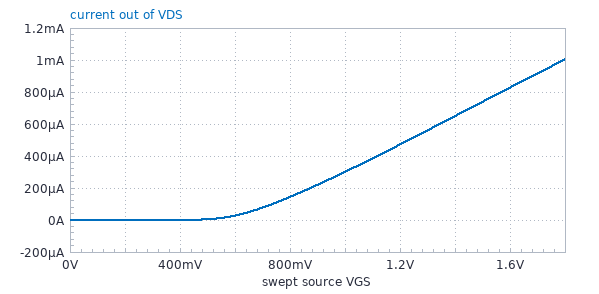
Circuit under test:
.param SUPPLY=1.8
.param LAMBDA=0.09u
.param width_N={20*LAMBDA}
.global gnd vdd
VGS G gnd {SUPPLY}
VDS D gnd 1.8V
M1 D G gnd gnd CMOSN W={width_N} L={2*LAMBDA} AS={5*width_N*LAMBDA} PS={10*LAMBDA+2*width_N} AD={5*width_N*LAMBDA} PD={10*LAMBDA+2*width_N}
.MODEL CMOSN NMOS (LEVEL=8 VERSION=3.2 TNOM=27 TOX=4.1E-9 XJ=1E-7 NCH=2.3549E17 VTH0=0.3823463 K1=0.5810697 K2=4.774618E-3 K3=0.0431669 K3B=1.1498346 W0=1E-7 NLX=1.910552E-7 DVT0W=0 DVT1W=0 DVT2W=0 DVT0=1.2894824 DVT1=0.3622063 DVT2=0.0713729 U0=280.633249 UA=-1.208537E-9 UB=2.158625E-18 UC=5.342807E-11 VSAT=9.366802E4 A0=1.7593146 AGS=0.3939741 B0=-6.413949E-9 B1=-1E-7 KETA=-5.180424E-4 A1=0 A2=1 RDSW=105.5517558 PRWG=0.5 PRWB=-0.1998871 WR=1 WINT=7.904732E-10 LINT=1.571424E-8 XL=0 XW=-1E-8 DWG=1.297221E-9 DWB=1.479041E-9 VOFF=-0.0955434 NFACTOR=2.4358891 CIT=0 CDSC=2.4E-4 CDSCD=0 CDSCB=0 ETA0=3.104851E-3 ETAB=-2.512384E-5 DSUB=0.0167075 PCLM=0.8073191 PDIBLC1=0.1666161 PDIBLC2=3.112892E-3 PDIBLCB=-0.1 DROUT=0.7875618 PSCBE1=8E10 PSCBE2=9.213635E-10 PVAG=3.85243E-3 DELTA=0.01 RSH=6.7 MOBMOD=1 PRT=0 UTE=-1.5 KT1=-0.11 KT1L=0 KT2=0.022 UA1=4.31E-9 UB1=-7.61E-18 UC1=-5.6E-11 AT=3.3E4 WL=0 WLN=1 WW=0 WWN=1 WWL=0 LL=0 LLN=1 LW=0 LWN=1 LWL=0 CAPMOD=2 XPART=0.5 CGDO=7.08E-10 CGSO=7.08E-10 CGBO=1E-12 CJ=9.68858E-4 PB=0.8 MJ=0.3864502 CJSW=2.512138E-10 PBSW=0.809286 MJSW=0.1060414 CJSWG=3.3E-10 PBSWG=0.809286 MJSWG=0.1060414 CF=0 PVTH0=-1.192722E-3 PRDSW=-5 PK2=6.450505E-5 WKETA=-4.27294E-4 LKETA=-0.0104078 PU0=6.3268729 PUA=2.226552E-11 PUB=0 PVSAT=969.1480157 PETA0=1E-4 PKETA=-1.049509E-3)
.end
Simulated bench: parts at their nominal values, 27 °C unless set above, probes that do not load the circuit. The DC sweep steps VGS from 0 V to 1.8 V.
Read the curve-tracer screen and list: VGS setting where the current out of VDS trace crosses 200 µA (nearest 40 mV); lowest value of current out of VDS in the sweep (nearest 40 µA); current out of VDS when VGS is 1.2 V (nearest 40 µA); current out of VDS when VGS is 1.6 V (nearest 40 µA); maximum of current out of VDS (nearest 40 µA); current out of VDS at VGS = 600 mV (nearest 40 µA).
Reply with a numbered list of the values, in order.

1. 880 mV
2. 0 A
3. 480 µA
4. 840 µA
5. 1.00 mA
6. 40 µA
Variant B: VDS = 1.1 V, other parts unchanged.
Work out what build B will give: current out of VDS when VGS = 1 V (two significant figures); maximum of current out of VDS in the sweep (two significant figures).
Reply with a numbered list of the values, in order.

1. 280 µA
2. 960 µA
